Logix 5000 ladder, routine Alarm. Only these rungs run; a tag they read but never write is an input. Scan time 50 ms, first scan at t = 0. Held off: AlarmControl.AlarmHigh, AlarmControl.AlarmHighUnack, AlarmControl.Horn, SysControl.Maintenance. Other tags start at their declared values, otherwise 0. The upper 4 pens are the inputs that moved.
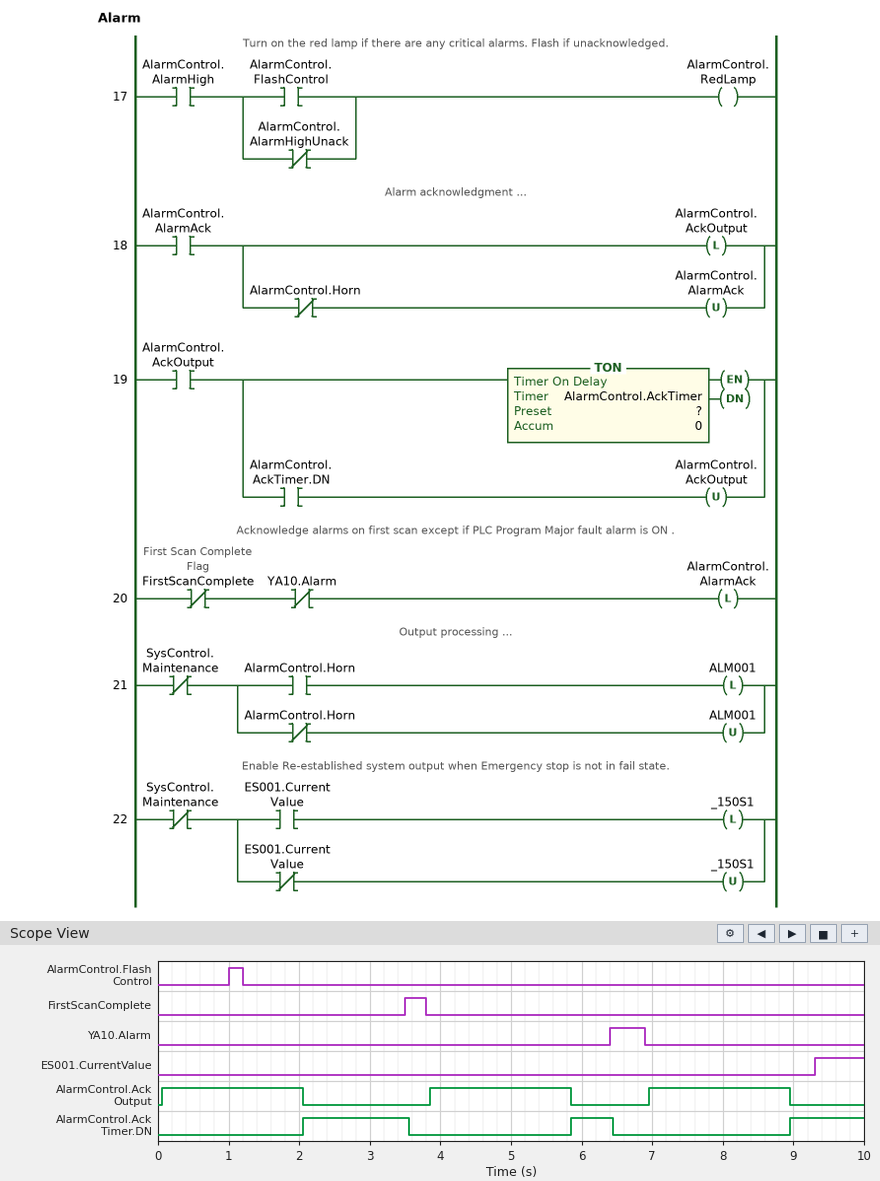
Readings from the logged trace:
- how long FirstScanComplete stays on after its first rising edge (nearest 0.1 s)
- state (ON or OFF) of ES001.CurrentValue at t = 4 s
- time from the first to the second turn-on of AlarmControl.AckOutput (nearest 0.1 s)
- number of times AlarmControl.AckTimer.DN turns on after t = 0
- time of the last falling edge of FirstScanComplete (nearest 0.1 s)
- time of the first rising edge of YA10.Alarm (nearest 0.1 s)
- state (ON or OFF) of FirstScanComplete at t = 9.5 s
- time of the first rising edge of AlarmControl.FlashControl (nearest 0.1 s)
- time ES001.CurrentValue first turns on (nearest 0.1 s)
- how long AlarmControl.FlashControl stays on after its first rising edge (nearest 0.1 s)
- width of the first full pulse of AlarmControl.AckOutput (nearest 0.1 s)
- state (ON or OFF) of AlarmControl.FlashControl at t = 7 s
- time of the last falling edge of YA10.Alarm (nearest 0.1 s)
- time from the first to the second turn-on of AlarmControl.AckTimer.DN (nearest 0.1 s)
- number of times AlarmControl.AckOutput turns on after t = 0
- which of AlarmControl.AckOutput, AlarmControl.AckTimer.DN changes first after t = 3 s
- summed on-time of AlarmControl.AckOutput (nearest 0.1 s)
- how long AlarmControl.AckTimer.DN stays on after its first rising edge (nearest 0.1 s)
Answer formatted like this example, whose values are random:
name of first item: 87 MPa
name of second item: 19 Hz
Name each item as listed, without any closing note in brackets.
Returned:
how long FirstScanComplete stays on after its first rising edge: 0.3 s
state (ON or OFF) of ES001.CurrentValue at t = 4 s: OFF
time from the first to the second turn-on of AlarmControl.AckOutput: 3.8 s
number of times AlarmControl.AckTimer.DN turns on after t = 0: 3
time of the last falling edge of FirstScanComplete: 3.8 s
time of the first rising edge of YA10.Alarm: 6.4 s
state (ON or OFF) of FirstScanComplete at t = 9.5 s: OFF
time of the first rising edge of AlarmControl.FlashControl: 1.0 s
time ES001.CurrentValue first turns on: 9.3 s
how long AlarmControl.FlashControl stays on after its first rising edge: 0.2 s
width of the first full pulse of AlarmControl.AckOutput: 2.0 s
state (ON or OFF) of AlarmControl.FlashControl at t = 7 s: OFF
time of the last falling edge of YA10.Alarm: 6.9 s
time from the first to the second turn-on of AlarmControl.AckTimer.DN: 3.8 s
number of times AlarmControl.AckOutput turns on after t = 0: 3
which of AlarmControl.AckOutput, AlarmControl.AckTimer.DN changes first after t = 3 s: AlarmControl.AckTimer.DN
summed on-time of AlarmControl.AckOutput: 6.0 s
how long AlarmControl.AckTimer.DN stays on after its first rising edge: 1.5 s
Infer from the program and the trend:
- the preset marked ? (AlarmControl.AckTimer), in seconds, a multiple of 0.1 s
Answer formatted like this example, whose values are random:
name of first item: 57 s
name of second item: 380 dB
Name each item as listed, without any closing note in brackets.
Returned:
the preset marked ? (AlarmControl.AckTimer), in seconds, a multiple of 0.1 s: 2.0 s
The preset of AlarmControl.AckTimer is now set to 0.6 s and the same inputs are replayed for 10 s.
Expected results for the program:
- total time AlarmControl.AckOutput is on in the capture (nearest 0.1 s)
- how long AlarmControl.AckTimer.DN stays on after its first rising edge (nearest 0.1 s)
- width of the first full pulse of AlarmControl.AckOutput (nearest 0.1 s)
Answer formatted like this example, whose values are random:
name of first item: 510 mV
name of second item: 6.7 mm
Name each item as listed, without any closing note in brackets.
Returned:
total time AlarmControl.AckOutput is on in the capture: 1.8 s
how long AlarmControl.AckTimer.DN stays on after its first rising edge: 2.9 s
width of the first full pulse of AlarmControl.AckOutput: 0.6 s
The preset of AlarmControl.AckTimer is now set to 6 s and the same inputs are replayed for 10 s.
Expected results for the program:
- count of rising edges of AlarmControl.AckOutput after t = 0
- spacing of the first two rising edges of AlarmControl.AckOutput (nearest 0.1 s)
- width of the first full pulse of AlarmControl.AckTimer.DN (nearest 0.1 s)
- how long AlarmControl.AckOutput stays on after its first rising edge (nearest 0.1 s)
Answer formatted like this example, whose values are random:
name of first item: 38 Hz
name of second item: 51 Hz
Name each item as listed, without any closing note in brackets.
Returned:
count of rising edges of AlarmControl.AckOutput after t = 0: 2
spacing of the first two rising edges of AlarmControl.AckOutput: 6.9 s
width of the first full pulse of AlarmControl.AckTimer.DN: 0.4 s
how long AlarmControl.AckOutput stays on after its first rising edge: 6.0 s
